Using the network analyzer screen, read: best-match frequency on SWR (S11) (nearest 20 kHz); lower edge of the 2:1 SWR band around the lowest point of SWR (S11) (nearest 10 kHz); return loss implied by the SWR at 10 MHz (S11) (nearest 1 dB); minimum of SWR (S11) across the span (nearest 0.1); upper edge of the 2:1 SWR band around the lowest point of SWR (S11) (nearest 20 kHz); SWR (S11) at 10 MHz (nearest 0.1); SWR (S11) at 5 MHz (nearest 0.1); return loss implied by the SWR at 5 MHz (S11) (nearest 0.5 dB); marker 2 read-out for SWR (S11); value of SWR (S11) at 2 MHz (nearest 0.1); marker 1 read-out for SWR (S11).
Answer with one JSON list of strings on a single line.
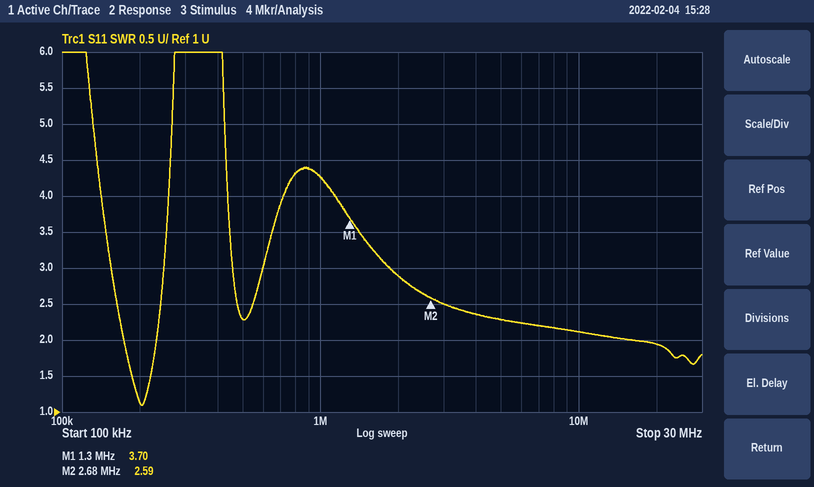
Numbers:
["200 kHz", "170 kHz", "9 dB", "1.1", "240 kHz", "2.1", "2.3", "8.0 dB", "2.59", "2.9", "3.70"]
